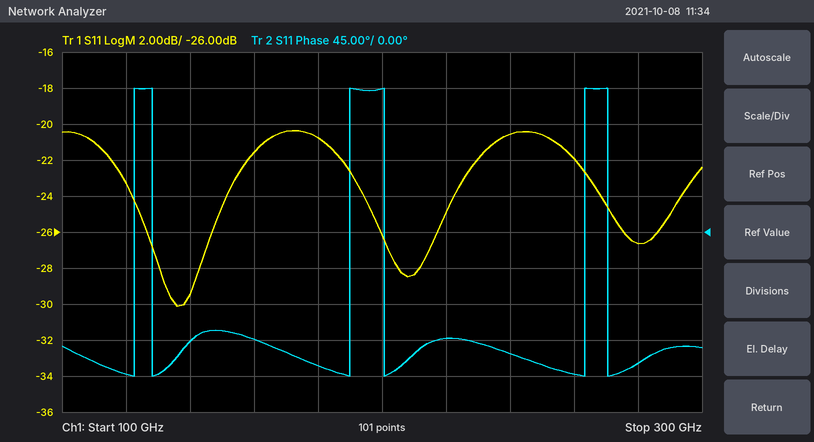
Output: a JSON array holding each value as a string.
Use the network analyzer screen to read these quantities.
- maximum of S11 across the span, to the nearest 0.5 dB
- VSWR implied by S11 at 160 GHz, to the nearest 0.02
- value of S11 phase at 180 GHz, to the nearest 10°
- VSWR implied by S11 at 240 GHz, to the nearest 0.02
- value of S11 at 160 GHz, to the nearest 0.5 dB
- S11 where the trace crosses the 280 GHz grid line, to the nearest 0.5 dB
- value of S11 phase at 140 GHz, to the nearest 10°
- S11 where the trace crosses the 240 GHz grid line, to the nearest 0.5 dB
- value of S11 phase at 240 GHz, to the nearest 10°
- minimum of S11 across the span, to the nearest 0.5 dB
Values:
["-20.5 dB", "1.18", "-170°", "1.20", "-21.5 dB", "-26.5 dB", "-140°", "-20.5 dB", "-150°", "-30.0 dB"]
